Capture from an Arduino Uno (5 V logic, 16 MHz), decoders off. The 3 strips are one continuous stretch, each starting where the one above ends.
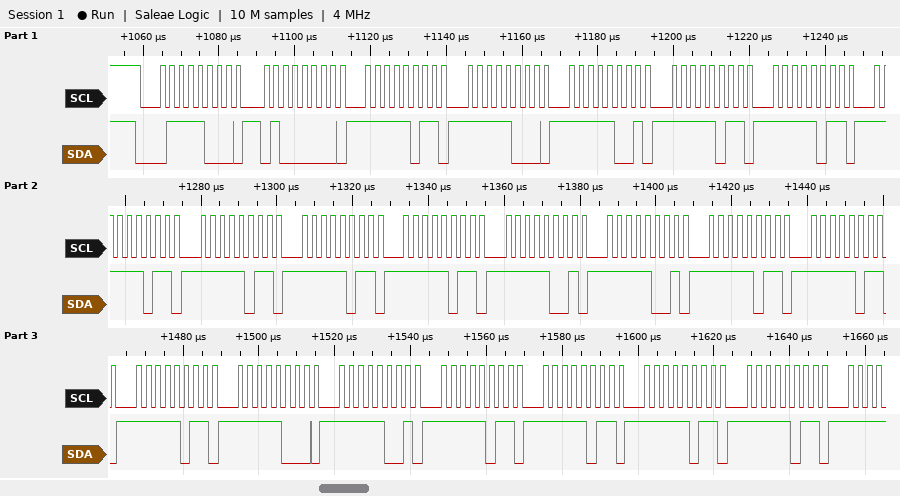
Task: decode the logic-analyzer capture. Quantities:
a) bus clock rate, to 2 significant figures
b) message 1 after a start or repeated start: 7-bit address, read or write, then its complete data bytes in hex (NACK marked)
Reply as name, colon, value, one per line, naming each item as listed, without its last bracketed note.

bus clock rate, to 2 significant figures: 400 kHz
message 1 after a start or repeated start: 7-bit address, read or write, then its complete data bytes in hex: 0x3C write: 40 FB F8 F9 FB FB FB FB FB FB F9 F9 FB FB FB F8 F9 FB FB FB FB
